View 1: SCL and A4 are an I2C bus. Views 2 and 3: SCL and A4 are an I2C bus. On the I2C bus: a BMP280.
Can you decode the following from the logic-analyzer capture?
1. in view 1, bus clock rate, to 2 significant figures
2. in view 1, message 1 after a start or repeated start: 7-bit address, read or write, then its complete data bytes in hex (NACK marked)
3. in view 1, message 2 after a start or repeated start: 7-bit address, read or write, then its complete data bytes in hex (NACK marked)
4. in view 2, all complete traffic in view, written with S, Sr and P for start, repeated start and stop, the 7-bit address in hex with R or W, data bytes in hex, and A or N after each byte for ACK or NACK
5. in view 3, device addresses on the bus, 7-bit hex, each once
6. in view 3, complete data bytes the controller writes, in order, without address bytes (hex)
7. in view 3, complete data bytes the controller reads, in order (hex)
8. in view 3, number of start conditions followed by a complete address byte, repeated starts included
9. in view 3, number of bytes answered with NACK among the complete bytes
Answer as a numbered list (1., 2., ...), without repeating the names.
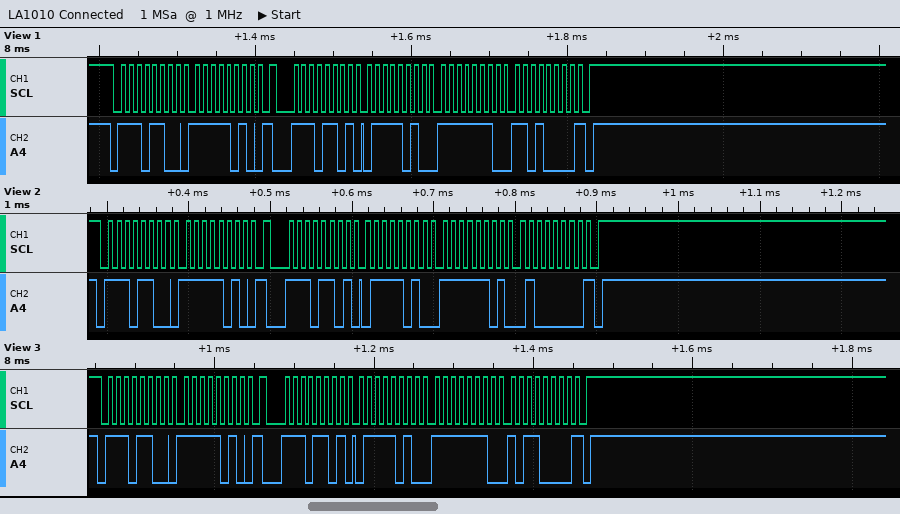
1. 100 kHz
2. 0x76 write: FA
3. 0x76 read: 7A FE D0 NACK
4. S 76W A FA A Sr 76R A 7A A FD A 40 N P
5. 0x76
6. FA
7. 7A FE B0
8. 2
9. 1
